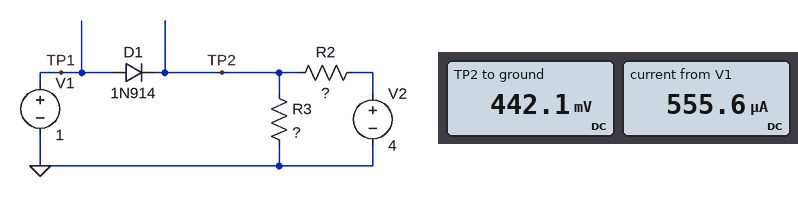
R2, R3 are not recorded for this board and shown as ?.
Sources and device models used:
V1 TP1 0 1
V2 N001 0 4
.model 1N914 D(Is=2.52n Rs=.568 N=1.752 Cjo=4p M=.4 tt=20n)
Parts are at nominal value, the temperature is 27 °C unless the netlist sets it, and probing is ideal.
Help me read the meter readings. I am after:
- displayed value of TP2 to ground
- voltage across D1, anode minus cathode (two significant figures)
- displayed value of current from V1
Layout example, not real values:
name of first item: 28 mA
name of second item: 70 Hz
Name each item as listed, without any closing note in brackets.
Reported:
displayed value of TP2 to ground: 442.1 mV
voltage across D1, anode minus cathode: 560 mV
displayed value of current from V1: 555.6 µA
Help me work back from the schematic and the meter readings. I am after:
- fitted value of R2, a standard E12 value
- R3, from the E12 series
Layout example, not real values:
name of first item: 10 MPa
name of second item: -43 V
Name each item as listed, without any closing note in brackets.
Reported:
fitted value of R2, a standard E12 value: 330 Ω
R3, from the E12 series: 39 Ω
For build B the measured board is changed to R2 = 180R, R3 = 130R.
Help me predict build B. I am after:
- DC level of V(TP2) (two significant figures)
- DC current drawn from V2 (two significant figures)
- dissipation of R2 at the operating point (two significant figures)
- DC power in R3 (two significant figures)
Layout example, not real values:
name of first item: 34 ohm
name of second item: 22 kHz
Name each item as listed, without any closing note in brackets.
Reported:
DC level of V(TP2): 1.7 V
DC current drawn from V2: 13 mA
dissipation of R2 at the operating point: 30 mW
DC power in R3: 22 mW
